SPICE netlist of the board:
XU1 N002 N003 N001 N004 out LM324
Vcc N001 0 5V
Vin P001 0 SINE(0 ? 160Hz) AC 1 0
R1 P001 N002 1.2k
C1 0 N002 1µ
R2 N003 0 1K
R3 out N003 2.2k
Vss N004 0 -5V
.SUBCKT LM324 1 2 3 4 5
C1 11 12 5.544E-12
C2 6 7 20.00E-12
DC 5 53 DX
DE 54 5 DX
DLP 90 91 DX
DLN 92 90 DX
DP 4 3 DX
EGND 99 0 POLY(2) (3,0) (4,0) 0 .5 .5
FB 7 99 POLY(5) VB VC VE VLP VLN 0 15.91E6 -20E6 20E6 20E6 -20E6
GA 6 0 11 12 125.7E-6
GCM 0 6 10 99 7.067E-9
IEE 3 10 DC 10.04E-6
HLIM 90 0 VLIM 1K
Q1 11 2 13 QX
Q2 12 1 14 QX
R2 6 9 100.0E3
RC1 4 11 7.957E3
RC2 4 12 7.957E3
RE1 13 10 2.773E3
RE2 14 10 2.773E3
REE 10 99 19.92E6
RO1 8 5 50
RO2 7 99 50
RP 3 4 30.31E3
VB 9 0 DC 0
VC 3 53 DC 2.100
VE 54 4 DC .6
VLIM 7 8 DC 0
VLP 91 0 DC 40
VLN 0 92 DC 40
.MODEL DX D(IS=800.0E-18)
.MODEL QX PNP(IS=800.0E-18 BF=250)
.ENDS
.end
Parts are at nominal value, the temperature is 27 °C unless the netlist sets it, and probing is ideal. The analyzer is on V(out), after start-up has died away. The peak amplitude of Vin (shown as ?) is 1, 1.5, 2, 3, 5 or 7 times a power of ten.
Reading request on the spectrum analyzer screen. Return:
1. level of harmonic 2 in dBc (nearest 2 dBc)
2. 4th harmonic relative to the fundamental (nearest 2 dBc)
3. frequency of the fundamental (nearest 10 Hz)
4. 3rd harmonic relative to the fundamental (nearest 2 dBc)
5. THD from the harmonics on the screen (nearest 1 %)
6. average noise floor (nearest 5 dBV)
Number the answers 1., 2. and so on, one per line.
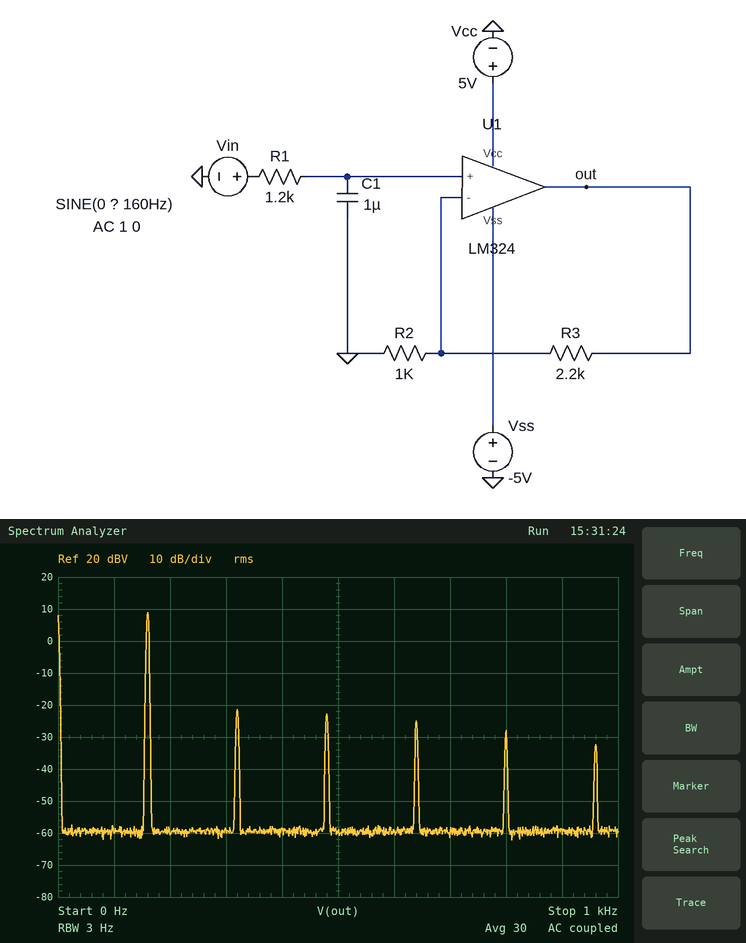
1. -30 dBc
2. -34 dBc
3. 160 Hz
4. -32 dBc
5. 5 %
6. -60 dBV
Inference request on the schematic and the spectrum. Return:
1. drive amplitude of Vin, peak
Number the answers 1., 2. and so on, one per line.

1. 2 V
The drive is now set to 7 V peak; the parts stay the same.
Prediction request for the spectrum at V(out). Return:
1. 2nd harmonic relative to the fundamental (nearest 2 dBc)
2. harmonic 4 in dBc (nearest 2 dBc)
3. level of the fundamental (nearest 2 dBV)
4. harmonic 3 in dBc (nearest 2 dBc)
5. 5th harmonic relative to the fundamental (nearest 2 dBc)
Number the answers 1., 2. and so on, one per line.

1. -26 dBc
2. -28 dBc
3. 12 dBV
4. -10 dBc
5. -18 dBc
